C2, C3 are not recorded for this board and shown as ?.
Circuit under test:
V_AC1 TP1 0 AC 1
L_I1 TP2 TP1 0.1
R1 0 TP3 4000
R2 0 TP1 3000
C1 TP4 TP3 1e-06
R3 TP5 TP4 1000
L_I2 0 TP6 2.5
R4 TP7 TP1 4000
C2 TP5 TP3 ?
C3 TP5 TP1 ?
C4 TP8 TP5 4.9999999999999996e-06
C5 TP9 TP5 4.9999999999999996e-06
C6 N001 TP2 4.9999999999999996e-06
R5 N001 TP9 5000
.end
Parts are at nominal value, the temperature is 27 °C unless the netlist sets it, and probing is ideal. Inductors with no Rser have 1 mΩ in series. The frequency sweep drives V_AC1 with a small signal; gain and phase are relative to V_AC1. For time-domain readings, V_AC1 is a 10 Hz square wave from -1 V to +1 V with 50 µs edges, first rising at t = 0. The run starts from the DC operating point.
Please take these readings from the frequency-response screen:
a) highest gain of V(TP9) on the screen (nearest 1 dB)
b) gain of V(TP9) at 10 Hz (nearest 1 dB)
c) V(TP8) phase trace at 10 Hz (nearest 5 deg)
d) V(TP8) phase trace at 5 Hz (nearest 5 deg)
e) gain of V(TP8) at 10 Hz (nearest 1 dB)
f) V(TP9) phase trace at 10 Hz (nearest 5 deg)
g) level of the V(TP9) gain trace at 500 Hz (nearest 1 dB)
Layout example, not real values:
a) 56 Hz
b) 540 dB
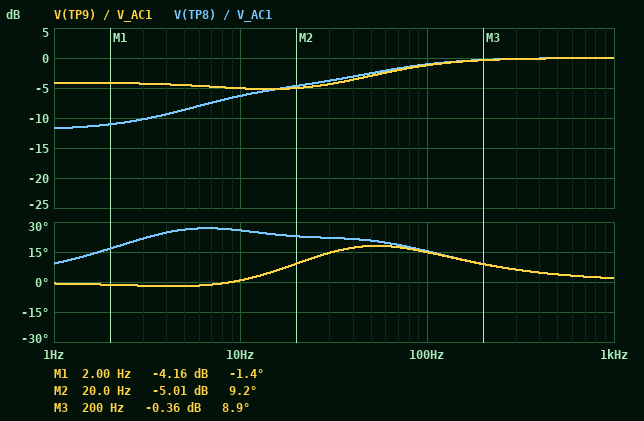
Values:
a) 0 dB
b) -5 dB
c) 25 deg
d) 25 deg
e) -6 dB
f) 0 deg
g) 0 dB
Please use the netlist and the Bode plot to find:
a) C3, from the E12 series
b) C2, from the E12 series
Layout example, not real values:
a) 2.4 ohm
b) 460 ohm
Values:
a) 1.2 µF
b) 10 µF
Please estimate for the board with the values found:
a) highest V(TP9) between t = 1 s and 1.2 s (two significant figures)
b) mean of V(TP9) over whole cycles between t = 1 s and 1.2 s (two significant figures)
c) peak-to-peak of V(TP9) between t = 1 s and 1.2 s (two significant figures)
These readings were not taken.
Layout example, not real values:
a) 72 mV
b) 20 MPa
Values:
a) 2.0 V
b) 630 mV
c) 2.8 V
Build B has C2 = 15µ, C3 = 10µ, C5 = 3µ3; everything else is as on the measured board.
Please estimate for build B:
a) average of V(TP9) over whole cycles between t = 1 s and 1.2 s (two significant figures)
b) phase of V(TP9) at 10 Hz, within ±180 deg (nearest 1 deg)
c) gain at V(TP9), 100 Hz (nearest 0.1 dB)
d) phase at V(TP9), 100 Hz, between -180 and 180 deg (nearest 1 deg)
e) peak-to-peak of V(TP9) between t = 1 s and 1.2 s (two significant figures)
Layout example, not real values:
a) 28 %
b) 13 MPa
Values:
a) 770 mV
b) 6 deg
c) -0.1 dB
d) 2 deg
e) 2.4 V
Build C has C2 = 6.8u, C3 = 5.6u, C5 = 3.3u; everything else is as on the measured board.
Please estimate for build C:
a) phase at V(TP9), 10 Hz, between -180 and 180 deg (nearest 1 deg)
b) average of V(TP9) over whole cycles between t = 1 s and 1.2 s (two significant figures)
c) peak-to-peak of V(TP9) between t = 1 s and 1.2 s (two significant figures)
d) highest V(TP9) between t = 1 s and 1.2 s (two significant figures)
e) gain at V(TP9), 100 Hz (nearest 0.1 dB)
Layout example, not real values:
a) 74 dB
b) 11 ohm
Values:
a) 4 deg
b) 800 mV
c) 2.4 V
d) 2.0 V
e) -0.1 dB
